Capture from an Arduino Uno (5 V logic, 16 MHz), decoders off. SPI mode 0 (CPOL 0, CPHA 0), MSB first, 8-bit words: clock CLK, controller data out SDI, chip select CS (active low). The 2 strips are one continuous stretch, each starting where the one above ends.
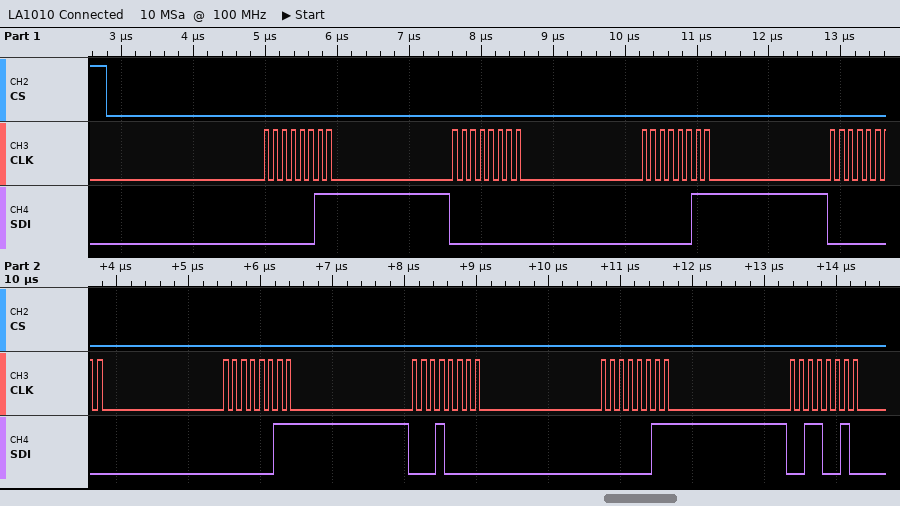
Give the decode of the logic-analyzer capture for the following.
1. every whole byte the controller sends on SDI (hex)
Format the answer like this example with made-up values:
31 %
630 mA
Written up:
03 00 03 00 03 10 03 32
